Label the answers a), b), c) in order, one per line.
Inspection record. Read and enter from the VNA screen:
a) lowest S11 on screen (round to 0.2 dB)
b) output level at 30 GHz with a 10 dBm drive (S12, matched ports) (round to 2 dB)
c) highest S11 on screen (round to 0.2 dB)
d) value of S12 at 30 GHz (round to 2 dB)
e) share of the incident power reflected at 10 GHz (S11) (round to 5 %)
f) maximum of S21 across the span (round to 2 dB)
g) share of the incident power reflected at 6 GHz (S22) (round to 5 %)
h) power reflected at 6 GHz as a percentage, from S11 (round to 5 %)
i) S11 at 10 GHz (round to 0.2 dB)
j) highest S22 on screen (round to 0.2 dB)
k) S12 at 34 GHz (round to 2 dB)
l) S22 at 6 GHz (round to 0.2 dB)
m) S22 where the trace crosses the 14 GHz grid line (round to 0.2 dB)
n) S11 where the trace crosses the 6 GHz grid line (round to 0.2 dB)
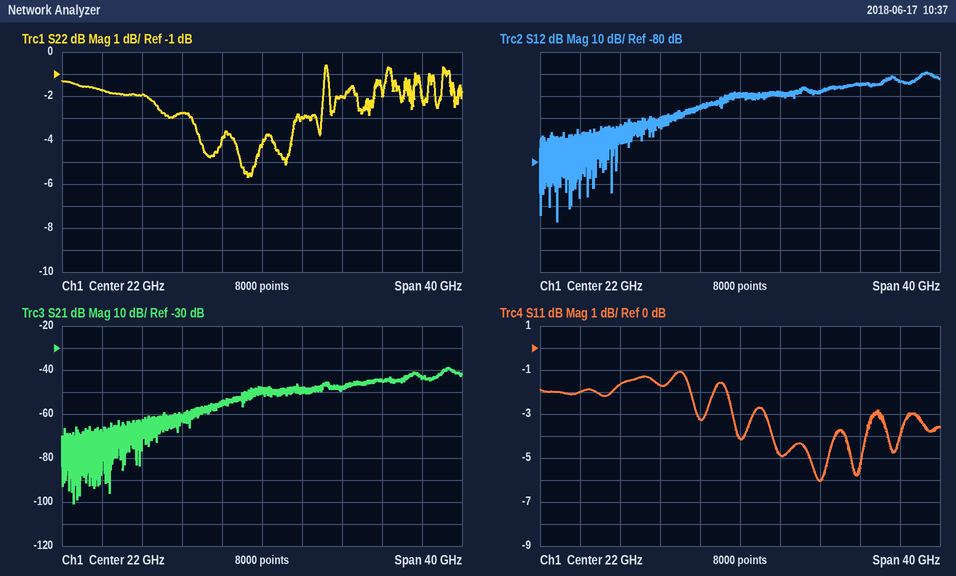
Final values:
a) -6.0 dB
b) -38 dBm
c) -1.0 dB
d) -48 dB
e) 70 %
f) -38 dB
g) 65 %
h) 65 %
i) -1.6 dB
j) -0.6 dB
k) -44 dB
l) -1.8 dB
m) -2.8 dB
n) -2.0 dB
